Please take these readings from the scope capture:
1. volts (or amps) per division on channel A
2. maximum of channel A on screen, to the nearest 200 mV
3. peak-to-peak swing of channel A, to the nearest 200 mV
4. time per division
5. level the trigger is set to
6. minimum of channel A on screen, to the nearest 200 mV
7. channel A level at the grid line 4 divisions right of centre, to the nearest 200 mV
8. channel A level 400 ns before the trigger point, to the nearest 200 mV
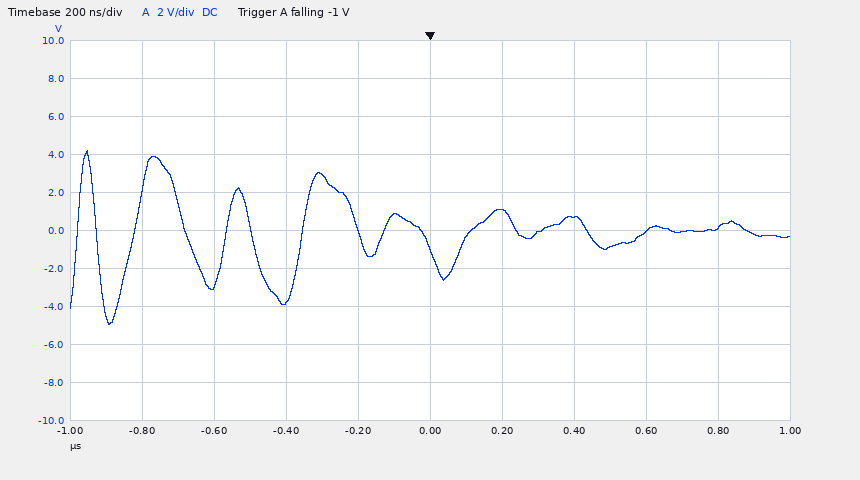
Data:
2 V
4.2 V
9.2 V
200 ns
-1 V
-5.0 V
200 mV
-3.8 V
